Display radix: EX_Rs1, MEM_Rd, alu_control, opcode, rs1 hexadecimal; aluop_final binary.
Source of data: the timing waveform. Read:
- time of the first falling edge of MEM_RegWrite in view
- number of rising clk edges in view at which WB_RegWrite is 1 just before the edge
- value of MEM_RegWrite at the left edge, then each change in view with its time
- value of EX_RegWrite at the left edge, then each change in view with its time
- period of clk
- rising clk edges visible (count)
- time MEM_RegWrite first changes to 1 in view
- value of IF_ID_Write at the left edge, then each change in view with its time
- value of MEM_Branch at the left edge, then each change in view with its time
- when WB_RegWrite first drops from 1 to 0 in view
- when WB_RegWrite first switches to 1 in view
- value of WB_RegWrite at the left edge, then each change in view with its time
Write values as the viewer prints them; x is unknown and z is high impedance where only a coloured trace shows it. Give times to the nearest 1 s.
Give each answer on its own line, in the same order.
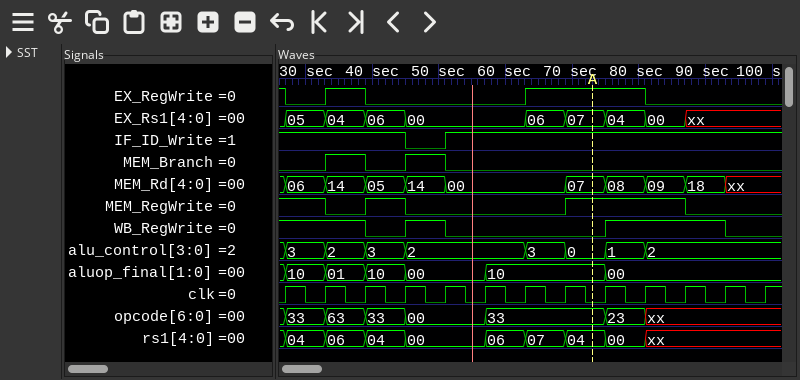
33 s
7
1, 0 at 33 s, 1 at 39 s, 0 at 45 s, 1 at 69 s, 0 at 87 s
1, 0 at 27 s, 1 at 33 s, 0 at 39 s, 1 at 63 s, 0 at 81 s
6 s
13
39 s
1, 0 at 45 s, 1 at 51 s
0, 1 at 33 s, 0 at 39 s, 1 at 45 s, 0 at 51 s
39 s
45 s
1, 0 at 39 s, 1 at 45 s, 0 at 51 s, 1 at 75 s, 0 at 93 s
